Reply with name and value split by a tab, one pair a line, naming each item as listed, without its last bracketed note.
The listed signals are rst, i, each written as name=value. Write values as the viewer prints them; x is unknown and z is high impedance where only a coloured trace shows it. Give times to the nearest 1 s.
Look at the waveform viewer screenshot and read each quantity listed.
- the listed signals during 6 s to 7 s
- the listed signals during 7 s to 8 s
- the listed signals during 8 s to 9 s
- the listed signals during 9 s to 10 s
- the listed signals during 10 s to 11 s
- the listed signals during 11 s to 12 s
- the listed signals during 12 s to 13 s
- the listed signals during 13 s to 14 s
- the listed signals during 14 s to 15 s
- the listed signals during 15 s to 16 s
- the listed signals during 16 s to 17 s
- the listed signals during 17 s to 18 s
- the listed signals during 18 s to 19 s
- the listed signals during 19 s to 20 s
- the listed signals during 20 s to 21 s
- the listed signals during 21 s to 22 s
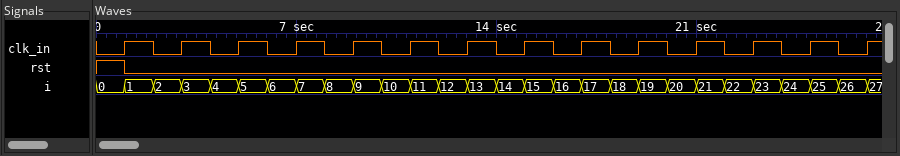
the listed signals during 6 s to 7 s	rst=0, i=6
the listed signals during 7 s to 8 s	rst=0, i=7
the listed signals during 8 s to 9 s	rst=0, i=8
the listed signals during 9 s to 10 s	rst=0, i=9
the listed signals during 10 s to 11 s	rst=0, i=10
the listed signals during 11 s to 12 s	rst=0, i=11
the listed signals during 12 s to 13 s	rst=0, i=12
the listed signals during 13 s to 14 s	rst=0, i=13
the listed signals during 14 s to 15 s	rst=0, i=14
the listed signals during 15 s to 16 s	rst=0, i=15
the listed signals during 16 s to 17 s	rst=0, i=16
the listed signals during 17 s to 18 s	rst=0, i=17
the listed signals during 18 s to 19 s	rst=0, i=18
the listed signals during 19 s to 20 s	rst=0, i=19
the listed signals during 20 s to 21 s	rst=0, i=20
the listed signals during 21 s to 22 s	rst=0, i=21
